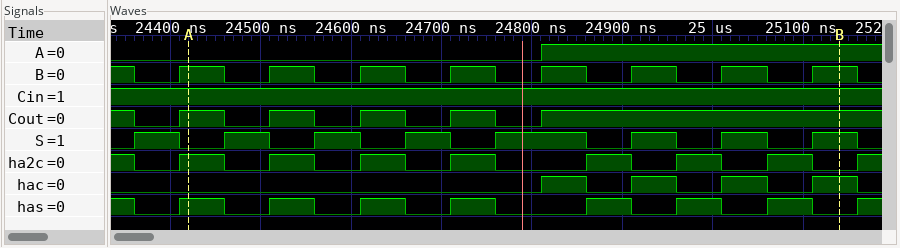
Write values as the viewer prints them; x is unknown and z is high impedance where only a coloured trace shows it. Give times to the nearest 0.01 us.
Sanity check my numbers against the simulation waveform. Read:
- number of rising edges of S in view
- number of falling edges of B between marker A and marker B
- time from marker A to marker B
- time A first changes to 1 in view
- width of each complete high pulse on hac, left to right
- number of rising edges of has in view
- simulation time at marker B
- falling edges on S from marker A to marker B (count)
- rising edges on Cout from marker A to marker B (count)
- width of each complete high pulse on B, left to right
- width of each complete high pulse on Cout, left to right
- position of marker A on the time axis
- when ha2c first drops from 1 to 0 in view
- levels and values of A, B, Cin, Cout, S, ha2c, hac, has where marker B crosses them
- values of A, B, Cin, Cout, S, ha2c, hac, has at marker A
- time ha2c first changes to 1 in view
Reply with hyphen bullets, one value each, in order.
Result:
- 8
- 7
- 0.72 us
- 24.81 us
- 0.05 us, 0.05 us, 0.05 us, 0.05 us
- 8
- 25.14 us
- 6
- 4
- 0.05 us, 0.05 us, 0.05 us, 0.05 us, 0.05 us, 0.05 us, 0.05 us, 0.05 us
- 0.05 us, 0.05 us, 0.05 us, 0.05 us
- 24.42 us
- 24.36 us
- A=1, B=1, Cin=1, Cout=1, S=1, ha2c=0, hac=1, has=0
- A=0, B=1, Cin=1, Cout=1, S=0, ha2c=1, hac=0, has=1
- 24.41 us
